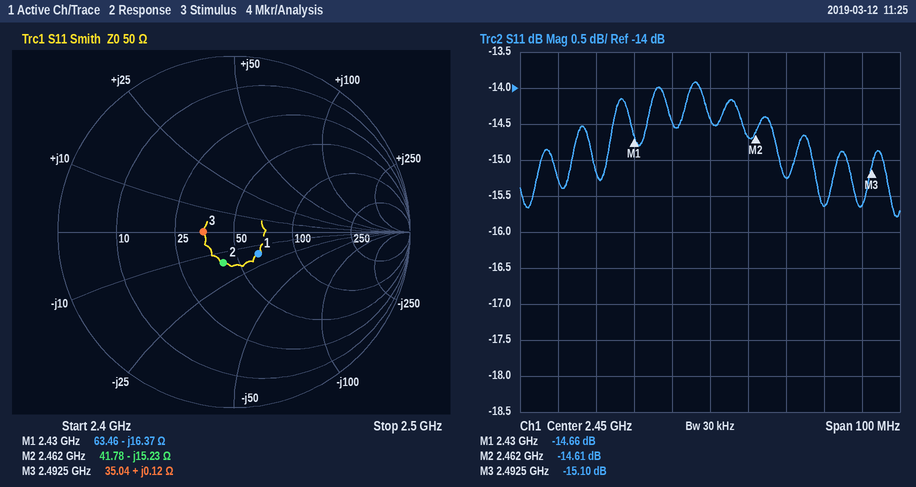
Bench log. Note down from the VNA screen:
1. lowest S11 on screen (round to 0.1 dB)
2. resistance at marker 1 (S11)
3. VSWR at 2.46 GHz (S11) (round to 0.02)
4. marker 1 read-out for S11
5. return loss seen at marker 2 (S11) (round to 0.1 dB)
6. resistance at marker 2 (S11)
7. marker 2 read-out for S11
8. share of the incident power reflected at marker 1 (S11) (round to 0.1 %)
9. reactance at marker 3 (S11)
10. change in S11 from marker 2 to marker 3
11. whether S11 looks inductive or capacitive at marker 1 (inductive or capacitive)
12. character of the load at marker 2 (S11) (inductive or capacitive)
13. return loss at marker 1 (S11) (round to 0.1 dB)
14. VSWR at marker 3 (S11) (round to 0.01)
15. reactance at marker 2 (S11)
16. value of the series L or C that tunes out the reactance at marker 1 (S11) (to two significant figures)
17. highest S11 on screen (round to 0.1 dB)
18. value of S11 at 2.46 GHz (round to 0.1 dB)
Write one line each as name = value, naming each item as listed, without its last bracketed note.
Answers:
lowest S11 on screen = -15.8 dB
resistance at marker 1 = 63.46 Ω
VSWR at 2.46 GHz (S11) = 1.46
marker 1 read-out for S11 = -14.66 dB
return loss seen at marker 2 (S11) = 14.6 dB
resistance at marker 2 = 41.78 Ω
marker 2 read-out for S11 = -14.61 dB
share of the incident power reflected at marker 1 (S11) = 3.4 %
reactance at marker 3 = +0.12 Ω
change in S11 from marker 2 to marker 3 = -0.49 dB
whether S11 looks inductive or capacitive at marker 1 = capacitive
character of the load at marker 2 (S11) = capacitive
return loss at marker 1 (S11) = 14.7 dB
VSWR at marker 3 (S11) = 1.43
reactance at marker 2 = -15.23 Ω
value of the series L or C that tunes out the reactance at marker 1 (S11) = 1.1 nH
highest S11 on screen = -13.9 dB
value of S11 at 2.46 GHz = -14.7 dB
